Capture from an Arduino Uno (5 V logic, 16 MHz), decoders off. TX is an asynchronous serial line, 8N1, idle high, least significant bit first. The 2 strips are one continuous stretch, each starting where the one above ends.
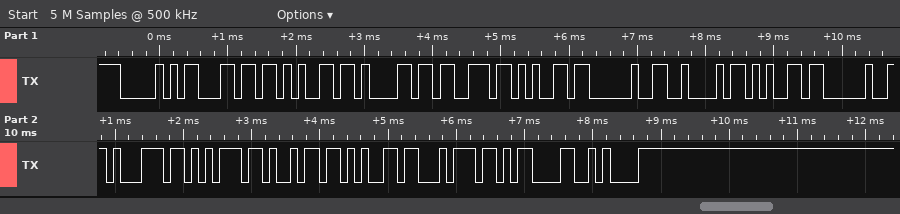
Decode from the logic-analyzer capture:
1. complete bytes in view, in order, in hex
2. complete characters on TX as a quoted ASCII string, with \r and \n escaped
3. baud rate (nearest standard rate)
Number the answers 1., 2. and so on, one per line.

1. 50 6C 65 61 73 65 20 42 65 20 71 75 69 65 74 0D 0A
2. "Please Be quiet\r\n"
3. 9600 baud
